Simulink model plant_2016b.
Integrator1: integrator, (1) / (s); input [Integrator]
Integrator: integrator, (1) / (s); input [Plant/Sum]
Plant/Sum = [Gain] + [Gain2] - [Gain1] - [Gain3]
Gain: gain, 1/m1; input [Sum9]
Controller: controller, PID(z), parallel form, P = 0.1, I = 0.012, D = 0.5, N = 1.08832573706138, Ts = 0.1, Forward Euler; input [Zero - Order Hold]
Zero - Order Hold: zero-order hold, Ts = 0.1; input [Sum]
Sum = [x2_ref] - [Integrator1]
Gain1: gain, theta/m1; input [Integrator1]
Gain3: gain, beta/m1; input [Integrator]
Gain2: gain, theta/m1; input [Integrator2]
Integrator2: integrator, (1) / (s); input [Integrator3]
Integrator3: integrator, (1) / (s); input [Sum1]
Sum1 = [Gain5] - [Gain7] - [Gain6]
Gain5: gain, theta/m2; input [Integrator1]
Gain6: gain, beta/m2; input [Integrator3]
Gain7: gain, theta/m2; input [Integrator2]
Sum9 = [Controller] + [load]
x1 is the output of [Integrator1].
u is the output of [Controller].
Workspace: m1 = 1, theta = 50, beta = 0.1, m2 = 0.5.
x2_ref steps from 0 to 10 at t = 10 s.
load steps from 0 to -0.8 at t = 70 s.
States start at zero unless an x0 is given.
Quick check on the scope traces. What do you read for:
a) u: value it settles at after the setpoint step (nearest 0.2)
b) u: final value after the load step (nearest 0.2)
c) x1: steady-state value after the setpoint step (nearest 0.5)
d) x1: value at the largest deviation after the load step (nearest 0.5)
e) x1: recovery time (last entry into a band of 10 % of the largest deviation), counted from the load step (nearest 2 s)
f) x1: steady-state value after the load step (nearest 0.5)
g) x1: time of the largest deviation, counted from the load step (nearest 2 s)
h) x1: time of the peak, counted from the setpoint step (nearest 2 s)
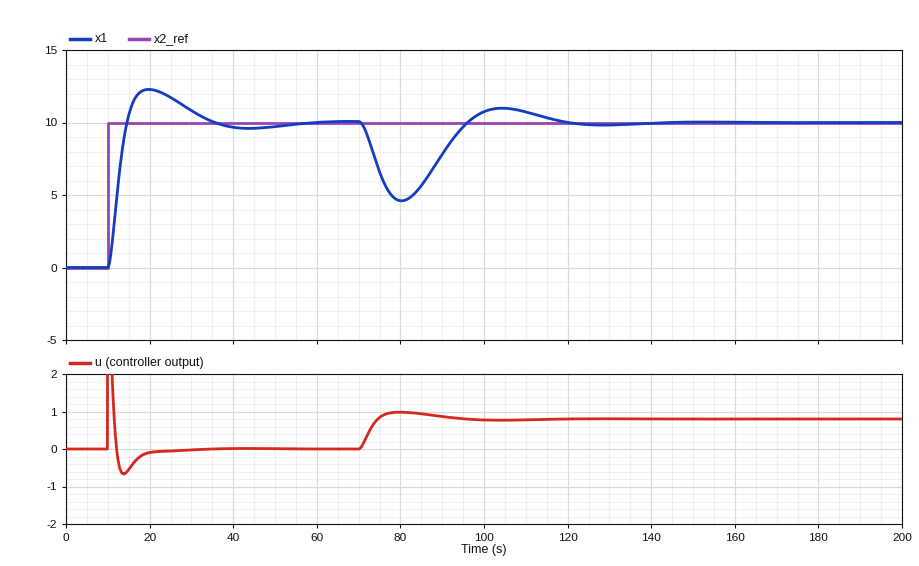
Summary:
0.0
0.8
10.0
4.5
42 s
10.0
10 s
10 s
